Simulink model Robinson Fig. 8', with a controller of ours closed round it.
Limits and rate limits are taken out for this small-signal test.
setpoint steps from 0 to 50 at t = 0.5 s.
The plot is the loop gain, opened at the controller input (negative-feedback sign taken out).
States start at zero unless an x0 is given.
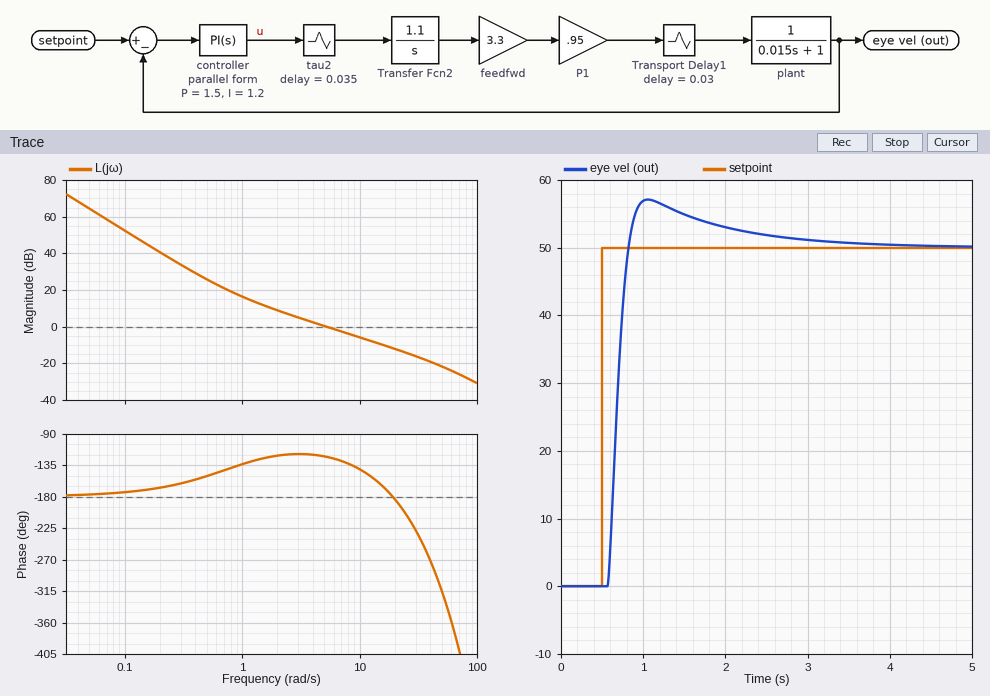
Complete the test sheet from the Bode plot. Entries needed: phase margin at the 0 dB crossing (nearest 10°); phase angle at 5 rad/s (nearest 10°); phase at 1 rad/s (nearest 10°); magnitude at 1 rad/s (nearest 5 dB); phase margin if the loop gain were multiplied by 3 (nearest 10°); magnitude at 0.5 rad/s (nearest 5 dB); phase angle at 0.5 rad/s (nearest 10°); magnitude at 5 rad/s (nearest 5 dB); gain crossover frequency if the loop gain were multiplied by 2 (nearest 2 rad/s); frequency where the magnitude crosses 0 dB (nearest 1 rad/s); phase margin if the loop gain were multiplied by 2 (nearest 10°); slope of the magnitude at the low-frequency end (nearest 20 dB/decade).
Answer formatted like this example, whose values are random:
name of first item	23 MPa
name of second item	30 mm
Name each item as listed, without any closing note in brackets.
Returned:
phase margin at the 0 dB crossing	60°
phase angle at 5 rad/s	-120°
phase at 1 rad/s	-130°
magnitude at 1 rad/s	15 dB
phase margin if the loop gain were multiplied by 3	20°
magnitude at 0.5 rad/s	25 dB
phase angle at 0.5 rad/s	-150°
magnitude at 5 rad/s	0 dB
gain crossover frequency if the loop gain were multiplied by 2	10 rad/s
frequency where the magnitude crosses 0 dB	5 rad/s
phase margin if the loop gain were multiplied by 2	40°
slope of the magnitude at the low-frequency end	-40 dB/decade
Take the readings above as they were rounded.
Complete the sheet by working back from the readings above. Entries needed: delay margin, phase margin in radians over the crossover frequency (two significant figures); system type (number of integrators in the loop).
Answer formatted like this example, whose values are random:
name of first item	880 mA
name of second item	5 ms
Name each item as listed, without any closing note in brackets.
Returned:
delay margin, phase margin in radians over the crossover frequency	0.21 s
system type	2
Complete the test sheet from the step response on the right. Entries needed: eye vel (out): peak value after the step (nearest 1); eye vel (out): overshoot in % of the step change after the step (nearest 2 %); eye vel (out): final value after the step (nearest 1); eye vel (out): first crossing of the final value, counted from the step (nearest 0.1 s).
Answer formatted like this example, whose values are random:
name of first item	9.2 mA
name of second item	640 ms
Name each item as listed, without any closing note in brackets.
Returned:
eye vel (out): peak value after the step	57
eye vel (out): overshoot in % of the step change after the step	14 %
eye vel (out): final value after the step	50
eye vel (out): first crossing of the final value, counted from the step	0.3 s
